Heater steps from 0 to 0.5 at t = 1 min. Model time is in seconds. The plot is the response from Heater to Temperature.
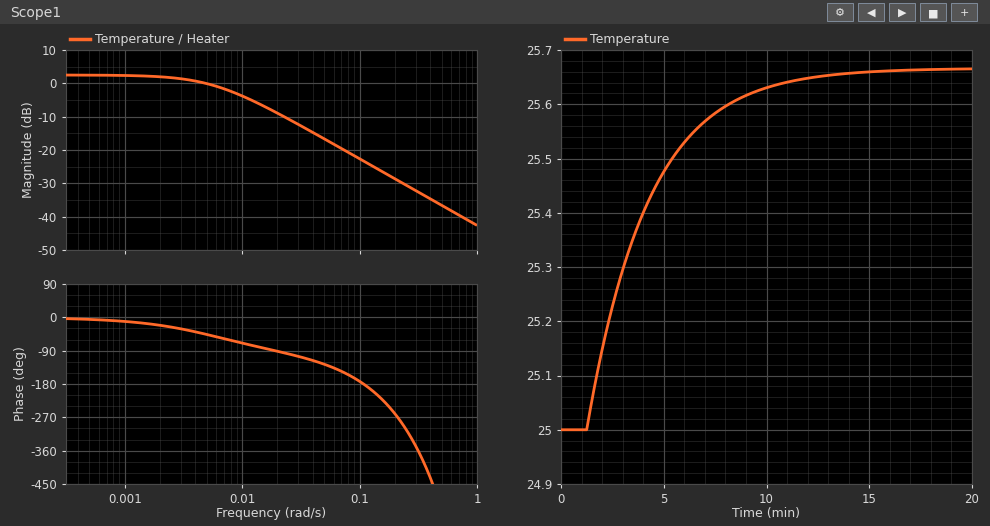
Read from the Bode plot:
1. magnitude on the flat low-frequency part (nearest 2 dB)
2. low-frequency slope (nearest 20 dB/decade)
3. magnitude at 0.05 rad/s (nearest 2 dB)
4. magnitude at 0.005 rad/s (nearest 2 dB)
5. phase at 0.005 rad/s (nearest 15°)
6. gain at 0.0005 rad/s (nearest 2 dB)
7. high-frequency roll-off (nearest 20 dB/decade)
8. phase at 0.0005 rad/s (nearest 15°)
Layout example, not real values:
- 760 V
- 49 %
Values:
- 2 dB
- 0 dB/decade
- -16 dB
- 0 dB
- -45°
- 2 dB
- -20 dB/decade
- 0°
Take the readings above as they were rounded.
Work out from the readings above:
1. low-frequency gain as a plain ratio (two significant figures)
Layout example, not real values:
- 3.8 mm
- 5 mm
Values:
- 1.3
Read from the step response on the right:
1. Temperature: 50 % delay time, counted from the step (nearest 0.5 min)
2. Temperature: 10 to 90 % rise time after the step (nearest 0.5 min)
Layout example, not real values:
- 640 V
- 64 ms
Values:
- 2.5 min
- 6.5 min
